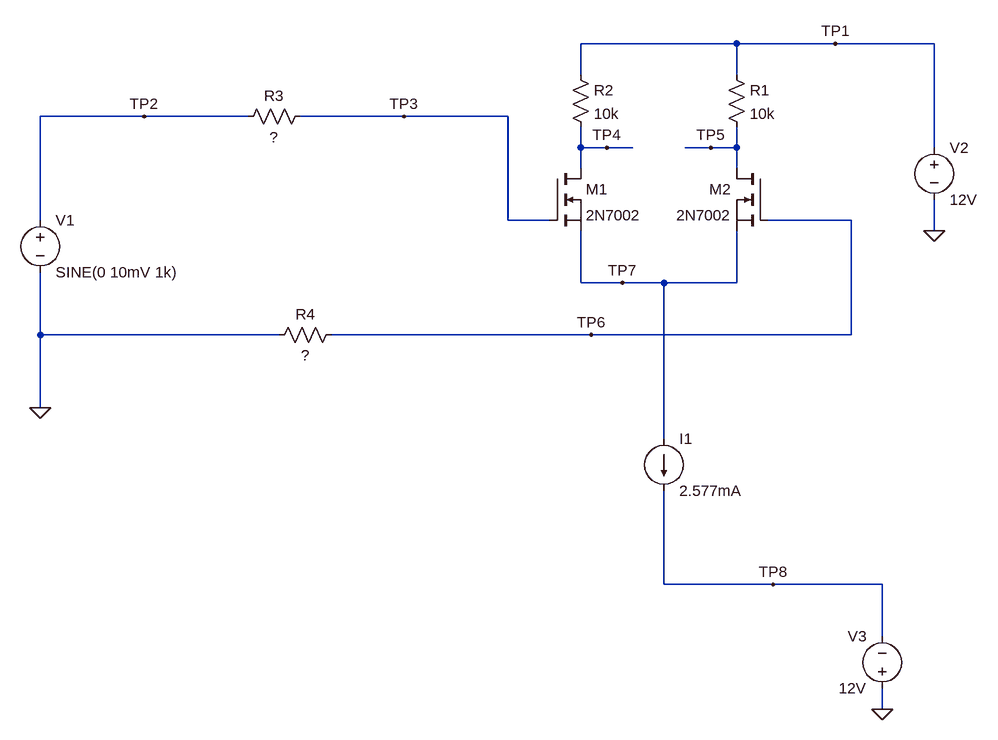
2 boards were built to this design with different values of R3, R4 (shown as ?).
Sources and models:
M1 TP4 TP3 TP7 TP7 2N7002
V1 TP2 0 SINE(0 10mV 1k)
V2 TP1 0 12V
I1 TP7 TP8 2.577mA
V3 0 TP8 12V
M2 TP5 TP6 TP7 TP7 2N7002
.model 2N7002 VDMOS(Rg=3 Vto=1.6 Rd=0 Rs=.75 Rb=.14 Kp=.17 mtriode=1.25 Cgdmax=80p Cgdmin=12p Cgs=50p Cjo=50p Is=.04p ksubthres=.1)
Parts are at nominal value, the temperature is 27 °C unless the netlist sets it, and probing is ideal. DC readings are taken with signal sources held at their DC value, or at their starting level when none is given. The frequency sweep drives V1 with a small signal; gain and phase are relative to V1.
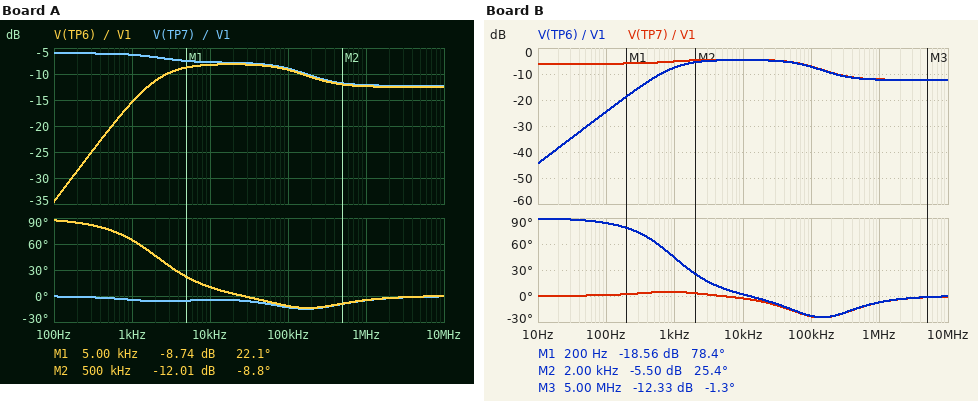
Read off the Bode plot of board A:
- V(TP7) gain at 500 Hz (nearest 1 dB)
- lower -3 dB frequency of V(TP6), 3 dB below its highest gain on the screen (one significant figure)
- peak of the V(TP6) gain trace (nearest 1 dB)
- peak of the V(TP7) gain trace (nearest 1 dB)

-6 dB
2 kHz
-8 dB
-6 dB
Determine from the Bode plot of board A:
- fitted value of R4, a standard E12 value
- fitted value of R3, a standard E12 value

5.6 kΩ
8.2 kΩ
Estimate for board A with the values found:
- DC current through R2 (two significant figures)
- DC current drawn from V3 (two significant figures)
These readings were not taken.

1.3 mA
2.6 mA
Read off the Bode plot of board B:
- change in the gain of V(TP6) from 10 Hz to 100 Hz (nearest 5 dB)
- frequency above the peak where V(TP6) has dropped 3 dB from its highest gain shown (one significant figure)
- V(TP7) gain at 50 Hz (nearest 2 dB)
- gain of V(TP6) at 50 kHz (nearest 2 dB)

20 dB
100 kHz
-6 dB
-6 dB
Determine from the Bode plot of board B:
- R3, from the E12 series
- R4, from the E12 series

12 kΩ
18 kΩ
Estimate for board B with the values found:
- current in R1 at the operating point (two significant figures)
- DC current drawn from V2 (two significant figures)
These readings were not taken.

1.3 mA
2.6 mA
